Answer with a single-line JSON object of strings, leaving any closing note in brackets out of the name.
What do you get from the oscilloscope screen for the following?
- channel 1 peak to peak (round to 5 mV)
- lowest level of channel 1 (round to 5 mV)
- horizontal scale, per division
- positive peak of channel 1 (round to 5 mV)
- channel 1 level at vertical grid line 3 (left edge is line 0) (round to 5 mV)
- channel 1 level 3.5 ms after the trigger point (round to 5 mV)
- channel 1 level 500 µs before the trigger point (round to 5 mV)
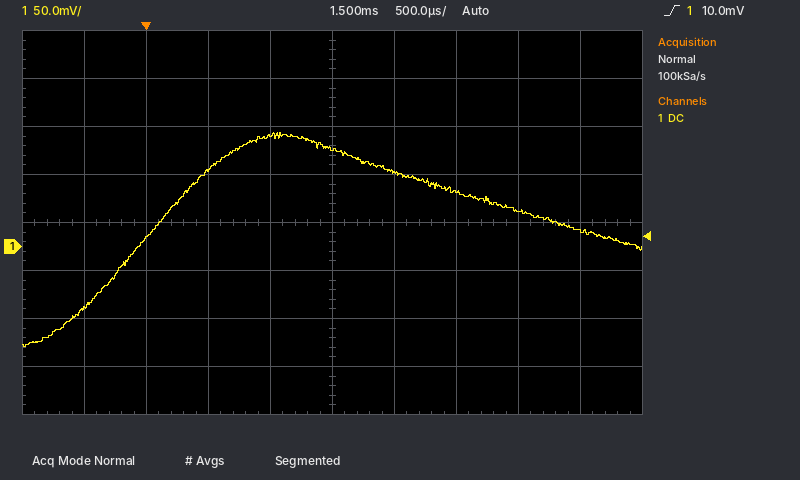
{"channel 1 peak to peak": "225 mV", "lowest level of channel 1": "-105 mV", "horizontal scale, per division": "500 µs", "positive peak of channel 1": "120 mV", "channel 1 level at vertical grid line 3 (left edge is line 0)": "80 mV", "channel 1 level 3.5 ms after the trigger point": "15 mV", "channel 1 level 500 µs before the trigger point": "-65 mV"}
